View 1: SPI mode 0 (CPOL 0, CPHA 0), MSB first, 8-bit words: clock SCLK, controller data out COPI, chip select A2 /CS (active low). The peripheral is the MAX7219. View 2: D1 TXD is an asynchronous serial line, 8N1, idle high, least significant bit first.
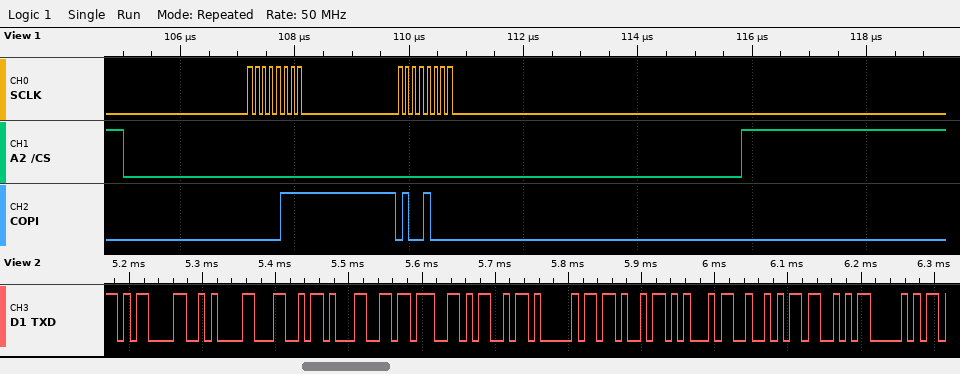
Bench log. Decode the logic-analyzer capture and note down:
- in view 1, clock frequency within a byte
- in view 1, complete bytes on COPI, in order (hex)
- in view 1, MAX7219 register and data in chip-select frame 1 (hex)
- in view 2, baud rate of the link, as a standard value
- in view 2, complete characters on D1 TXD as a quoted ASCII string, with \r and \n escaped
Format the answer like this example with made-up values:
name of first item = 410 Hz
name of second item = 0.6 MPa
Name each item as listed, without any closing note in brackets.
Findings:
in view 1, clock frequency within a byte = 8 MHz
in view 1, complete bytes on COPI, in order = 07 48
in view 1, MAX7219 register and data in chip-select frame 1 = register 0x7, data 0x48
in view 2, baud rate of the link, as a standard value = 115200 baud
in view 2, complete characters on D1 TXD as a quoted ASCII string, with \r and \n escaped = "\r\nL1;MAKERSP"
